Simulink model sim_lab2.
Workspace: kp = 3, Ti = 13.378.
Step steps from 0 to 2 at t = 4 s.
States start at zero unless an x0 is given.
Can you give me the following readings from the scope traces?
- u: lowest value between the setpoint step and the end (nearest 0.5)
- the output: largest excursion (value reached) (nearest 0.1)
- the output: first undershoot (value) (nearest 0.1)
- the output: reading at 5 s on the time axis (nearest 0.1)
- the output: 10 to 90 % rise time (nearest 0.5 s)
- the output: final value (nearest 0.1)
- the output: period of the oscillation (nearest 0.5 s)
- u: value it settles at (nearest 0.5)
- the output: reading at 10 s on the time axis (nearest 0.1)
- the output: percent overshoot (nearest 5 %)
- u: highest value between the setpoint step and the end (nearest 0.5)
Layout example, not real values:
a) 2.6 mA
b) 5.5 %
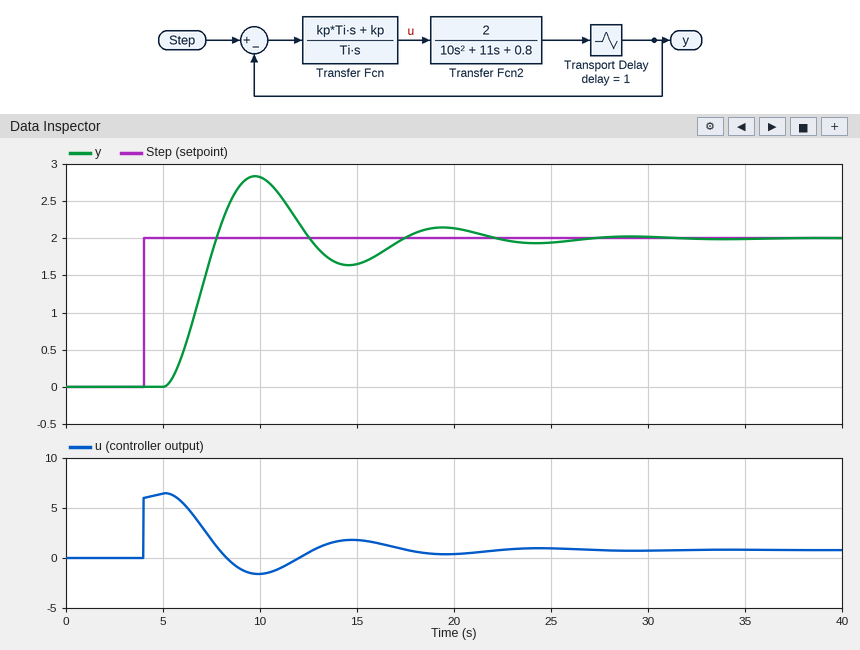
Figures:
a) -1.5
b) 2.8
c) 1.6
d) 0.0
e) 2.0 s
f) 2.0
g) 9.5 s
h) 1.0
i) 2.8
j) 40 %
k) 6.5
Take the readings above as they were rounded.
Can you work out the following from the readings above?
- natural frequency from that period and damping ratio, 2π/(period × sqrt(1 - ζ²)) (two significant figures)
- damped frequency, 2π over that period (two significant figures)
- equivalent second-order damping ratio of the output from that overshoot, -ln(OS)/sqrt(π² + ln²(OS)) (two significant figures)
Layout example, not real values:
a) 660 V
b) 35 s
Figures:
a) 0.69 rad/s
b) 0.66 rad/s
c) 0.28
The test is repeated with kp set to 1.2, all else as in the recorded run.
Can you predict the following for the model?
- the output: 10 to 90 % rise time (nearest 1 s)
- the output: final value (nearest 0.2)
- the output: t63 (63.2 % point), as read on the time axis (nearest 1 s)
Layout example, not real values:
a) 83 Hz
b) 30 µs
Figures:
a) 5 s
b) 2.0
c) 9 s
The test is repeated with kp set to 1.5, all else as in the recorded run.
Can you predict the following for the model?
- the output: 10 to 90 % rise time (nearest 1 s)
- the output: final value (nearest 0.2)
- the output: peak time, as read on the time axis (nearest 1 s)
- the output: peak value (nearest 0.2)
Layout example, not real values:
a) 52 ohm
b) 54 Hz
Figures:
a) 4 s
b) 2.0
c) 13 s
d) 2.2
